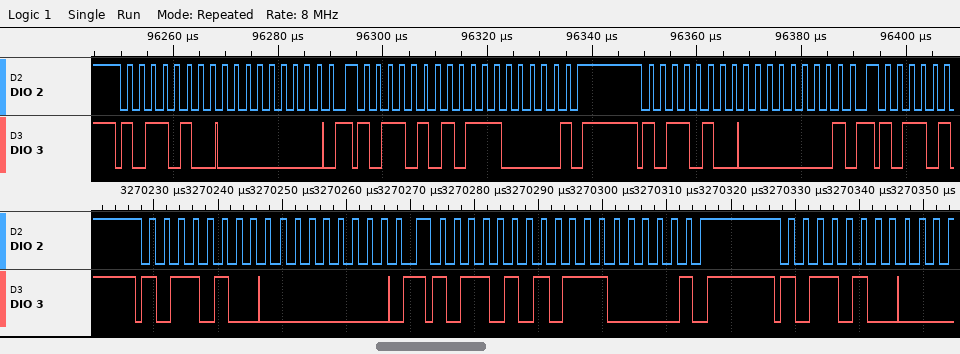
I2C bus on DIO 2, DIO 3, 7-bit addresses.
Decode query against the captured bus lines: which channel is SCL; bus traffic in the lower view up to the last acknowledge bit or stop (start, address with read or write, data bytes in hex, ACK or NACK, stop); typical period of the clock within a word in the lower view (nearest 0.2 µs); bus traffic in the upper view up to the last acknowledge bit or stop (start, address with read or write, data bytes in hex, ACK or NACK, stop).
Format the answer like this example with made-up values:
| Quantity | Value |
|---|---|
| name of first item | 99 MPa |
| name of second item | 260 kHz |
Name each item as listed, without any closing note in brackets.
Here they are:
| Quantity | Value |
|---|---|
| which channel is SCL | DIO 2 |
| bus traffic in the lower view up to the last acknowledge bit or stop | start, address 5A write ACK, 00 ACK, repeated start, address 5A read ACK, E0 NACK, stop, start, address 5A write ACK |
| typical period of the clock within a word in the lower view | 2.2 µs |
| bus traffic in the upper view up to the last acknowledge bit or stop | start, address 5A write ACK, 00 ACK, repeated start, address 5A read ACK, E0 NACK, stop, start, address 5A write ACK, 01 ACK |
